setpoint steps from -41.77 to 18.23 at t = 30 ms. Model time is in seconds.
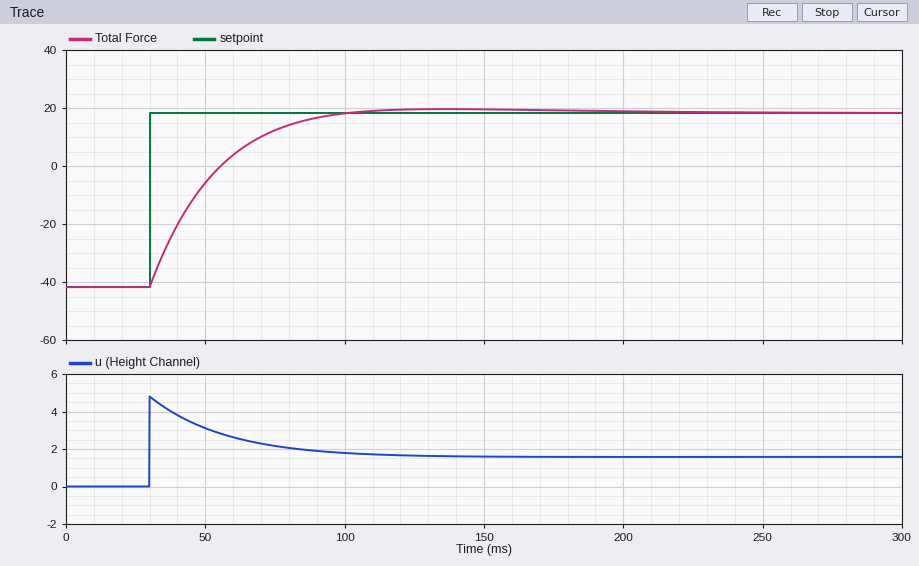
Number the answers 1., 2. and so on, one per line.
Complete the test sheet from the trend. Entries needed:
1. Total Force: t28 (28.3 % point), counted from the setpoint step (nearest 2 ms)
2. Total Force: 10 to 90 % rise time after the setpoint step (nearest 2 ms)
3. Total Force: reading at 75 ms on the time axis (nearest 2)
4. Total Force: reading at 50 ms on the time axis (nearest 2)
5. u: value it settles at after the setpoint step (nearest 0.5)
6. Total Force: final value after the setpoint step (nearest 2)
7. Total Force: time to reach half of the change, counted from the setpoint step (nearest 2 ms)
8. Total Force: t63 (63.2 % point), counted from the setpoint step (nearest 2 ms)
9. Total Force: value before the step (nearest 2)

1. 8 ms
2. 42 ms
3. 12
4. -6
5. 1.5
6. 18
7. 16 ms
8. 22 ms
9. -42
